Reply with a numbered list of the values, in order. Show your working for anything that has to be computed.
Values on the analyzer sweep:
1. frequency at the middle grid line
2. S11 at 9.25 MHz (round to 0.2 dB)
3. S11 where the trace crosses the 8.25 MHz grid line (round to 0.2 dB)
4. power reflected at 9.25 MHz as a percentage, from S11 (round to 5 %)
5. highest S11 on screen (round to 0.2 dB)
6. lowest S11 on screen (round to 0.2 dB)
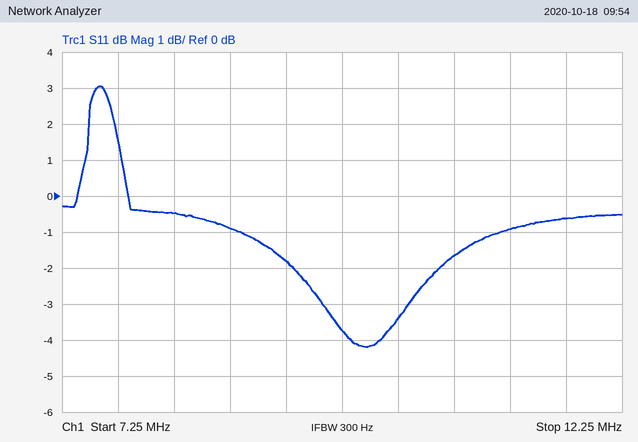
1. 9.75 MHz
2. -1.8 dB
3. -0.4 dB
4. 10^(-1.8/10) ≈ 66.1 %, so 65 % to the nearest 5 %
5. 3.0 dB
6. -4.2 dB
